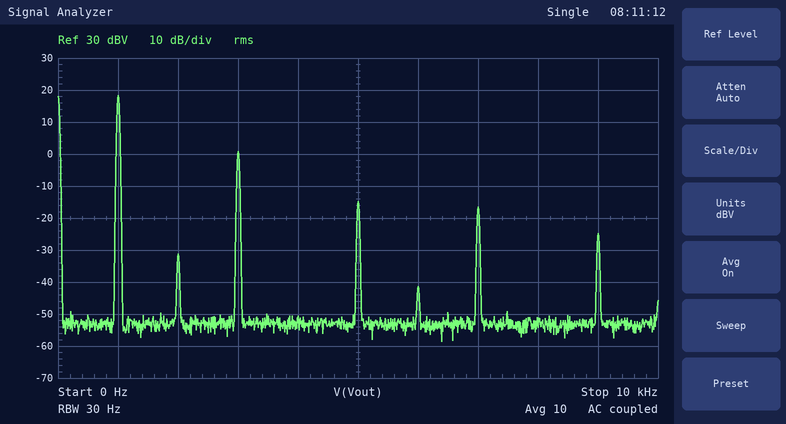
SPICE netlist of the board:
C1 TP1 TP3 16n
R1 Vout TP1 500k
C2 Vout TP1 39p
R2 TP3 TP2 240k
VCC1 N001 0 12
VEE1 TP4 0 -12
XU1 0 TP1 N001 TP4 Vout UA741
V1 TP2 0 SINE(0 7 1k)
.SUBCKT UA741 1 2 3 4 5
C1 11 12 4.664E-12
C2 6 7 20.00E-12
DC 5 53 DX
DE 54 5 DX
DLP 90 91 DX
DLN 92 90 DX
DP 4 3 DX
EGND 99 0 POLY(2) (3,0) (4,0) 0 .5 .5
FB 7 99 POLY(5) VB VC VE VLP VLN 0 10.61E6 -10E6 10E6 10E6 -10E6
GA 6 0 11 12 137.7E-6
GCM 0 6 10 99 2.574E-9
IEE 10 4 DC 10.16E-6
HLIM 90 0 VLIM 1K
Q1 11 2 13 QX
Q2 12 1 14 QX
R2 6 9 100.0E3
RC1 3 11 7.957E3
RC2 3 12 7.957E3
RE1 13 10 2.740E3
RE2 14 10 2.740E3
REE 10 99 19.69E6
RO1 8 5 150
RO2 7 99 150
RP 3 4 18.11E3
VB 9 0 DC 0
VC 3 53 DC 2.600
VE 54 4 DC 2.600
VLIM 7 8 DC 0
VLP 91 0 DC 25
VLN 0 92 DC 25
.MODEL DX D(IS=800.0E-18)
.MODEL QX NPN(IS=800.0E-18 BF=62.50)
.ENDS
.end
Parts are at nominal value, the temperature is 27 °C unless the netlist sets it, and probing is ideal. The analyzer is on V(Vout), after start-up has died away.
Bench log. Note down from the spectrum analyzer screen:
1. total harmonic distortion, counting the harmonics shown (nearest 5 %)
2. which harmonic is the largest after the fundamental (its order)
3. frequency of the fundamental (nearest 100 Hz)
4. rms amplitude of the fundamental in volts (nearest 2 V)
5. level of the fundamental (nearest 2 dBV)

15 %
3
1.0 kHz
8 V
18 dBV
